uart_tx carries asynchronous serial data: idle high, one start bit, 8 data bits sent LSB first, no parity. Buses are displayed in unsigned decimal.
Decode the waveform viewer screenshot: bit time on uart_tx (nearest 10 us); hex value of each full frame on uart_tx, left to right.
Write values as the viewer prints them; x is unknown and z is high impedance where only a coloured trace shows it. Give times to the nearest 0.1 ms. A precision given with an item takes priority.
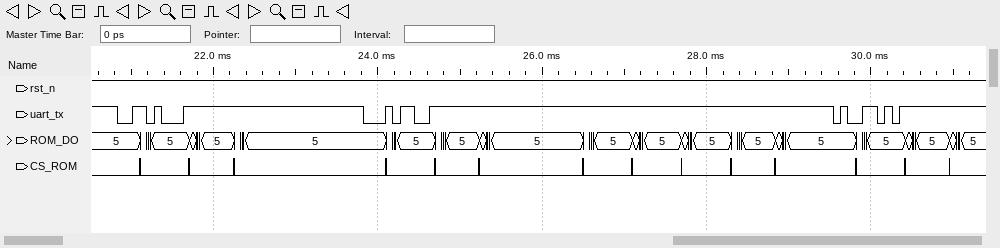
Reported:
90 us
16, 34, 59
